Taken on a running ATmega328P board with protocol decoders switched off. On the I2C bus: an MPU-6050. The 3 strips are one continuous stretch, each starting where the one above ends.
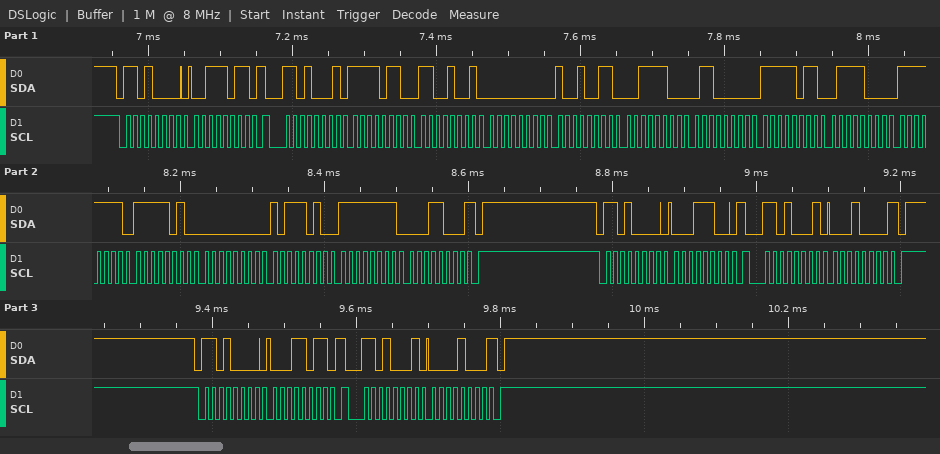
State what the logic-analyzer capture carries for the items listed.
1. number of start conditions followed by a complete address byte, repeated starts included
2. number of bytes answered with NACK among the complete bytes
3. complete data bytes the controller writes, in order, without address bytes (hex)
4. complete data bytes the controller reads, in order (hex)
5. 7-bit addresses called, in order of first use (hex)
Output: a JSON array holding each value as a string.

["6", "3", "3B 1C 1B", "F6 C9 00 93 3C 60 FB 78 FF FA 00 BA FF 18 10 08", "0x68"]
